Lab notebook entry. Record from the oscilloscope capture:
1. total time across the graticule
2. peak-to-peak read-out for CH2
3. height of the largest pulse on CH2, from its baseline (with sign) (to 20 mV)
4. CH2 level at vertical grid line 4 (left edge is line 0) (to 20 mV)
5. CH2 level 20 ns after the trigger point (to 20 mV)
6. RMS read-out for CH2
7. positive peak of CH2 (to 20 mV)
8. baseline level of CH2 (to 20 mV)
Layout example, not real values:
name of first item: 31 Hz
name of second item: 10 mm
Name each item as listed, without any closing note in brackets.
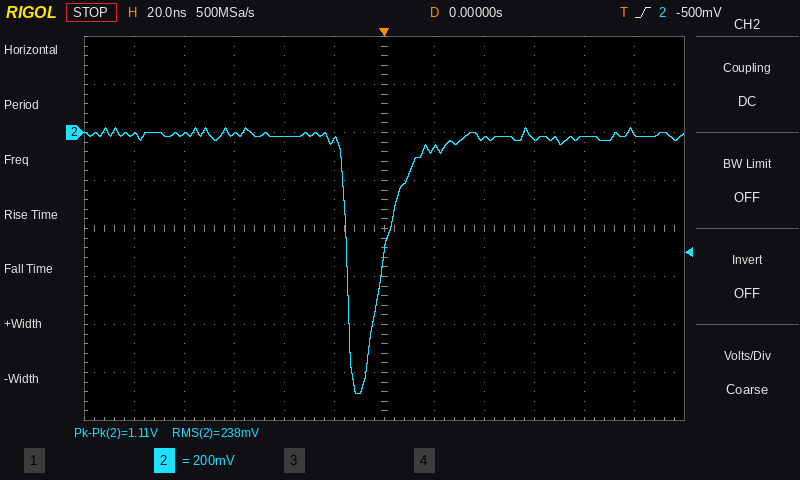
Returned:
total time across the graticule: 240 ns
peak-to-peak read-out for CH2: 1.11 V
height of the largest pulse on CH2, from its baseline (with sign): -1.08 V
CH2 level at vertical grid line 4 (left edge is line 0): -20 mV
CH2 level 20 ns after the trigger point: -60 mV
RMS read-out for CH2: 238 mV
positive peak of CH2: 20 mV
baseline level of CH2: -20 mV
